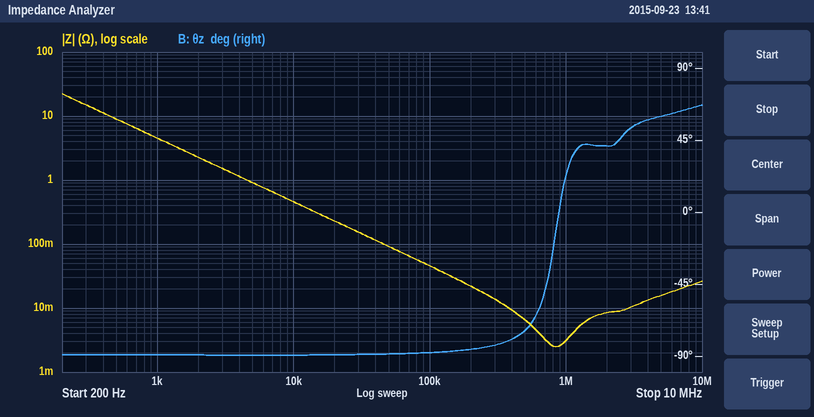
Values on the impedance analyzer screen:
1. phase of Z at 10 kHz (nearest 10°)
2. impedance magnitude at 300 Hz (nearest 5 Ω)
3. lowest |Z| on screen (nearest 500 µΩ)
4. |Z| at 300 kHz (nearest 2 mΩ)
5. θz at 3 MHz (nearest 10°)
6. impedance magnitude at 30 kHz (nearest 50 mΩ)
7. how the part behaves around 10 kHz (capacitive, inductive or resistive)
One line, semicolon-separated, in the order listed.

-90°; 15 Ω; 2.5 mΩ; 14 mΩ; 50°; 150 mΩ; capacitive
